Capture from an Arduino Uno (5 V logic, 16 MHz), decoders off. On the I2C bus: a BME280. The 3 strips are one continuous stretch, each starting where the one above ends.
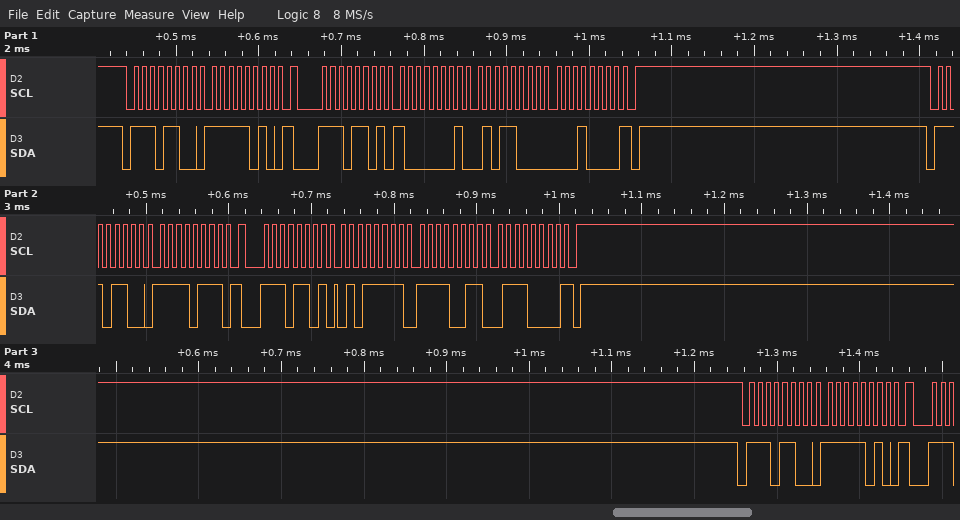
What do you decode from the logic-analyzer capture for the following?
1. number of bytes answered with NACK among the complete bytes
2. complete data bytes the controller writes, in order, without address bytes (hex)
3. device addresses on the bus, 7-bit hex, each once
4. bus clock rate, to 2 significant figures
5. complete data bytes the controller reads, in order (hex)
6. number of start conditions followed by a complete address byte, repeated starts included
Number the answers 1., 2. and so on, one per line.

1. 2
2. FA F7 FA
3. 0x76
4. 100 kHz
5. 81 58 10 5F F3 70
6. 5
